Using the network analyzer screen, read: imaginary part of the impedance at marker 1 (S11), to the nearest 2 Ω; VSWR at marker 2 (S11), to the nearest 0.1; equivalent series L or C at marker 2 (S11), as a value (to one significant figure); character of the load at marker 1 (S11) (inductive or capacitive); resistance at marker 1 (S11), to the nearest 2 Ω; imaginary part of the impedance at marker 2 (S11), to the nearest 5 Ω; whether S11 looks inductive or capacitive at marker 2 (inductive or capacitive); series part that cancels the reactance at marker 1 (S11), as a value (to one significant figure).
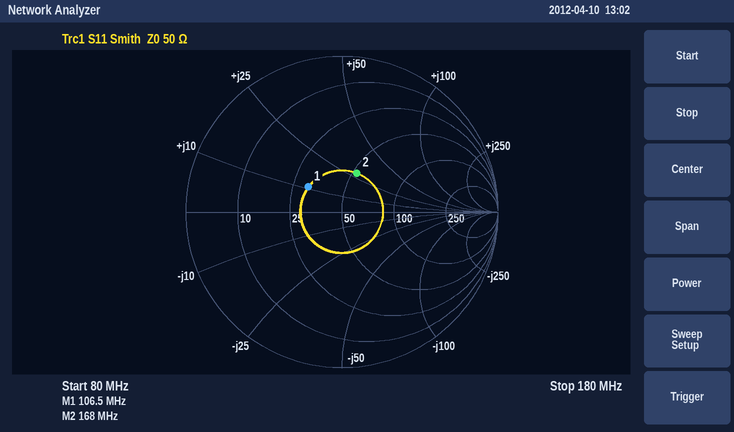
+10 Ω
1.7
30 nH
inductive
30 Ω
+30 Ω
inductive
100 pF
